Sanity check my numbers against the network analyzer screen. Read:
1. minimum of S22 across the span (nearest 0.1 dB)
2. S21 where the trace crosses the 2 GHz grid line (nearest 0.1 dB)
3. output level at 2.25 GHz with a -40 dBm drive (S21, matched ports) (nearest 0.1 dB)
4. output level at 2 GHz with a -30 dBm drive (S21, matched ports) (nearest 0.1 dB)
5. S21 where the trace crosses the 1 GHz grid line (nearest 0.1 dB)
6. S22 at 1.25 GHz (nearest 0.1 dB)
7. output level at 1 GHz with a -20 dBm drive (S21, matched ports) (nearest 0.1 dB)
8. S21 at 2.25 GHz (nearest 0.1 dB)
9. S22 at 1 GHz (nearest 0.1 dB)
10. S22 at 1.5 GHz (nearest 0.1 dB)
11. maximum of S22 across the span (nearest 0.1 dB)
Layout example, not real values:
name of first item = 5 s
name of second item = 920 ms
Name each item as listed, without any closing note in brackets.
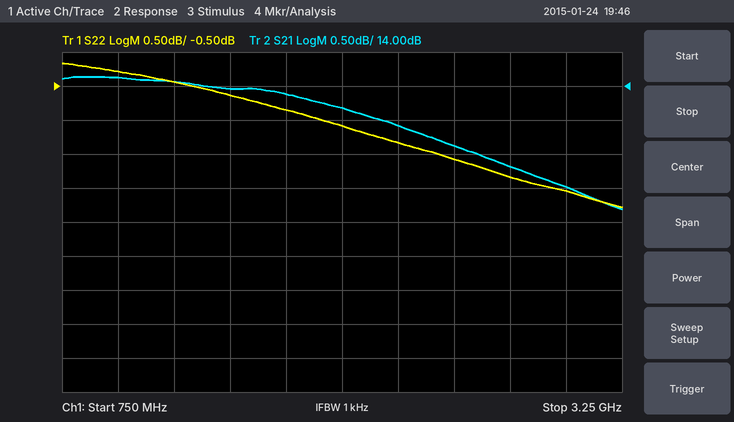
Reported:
minimum of S22 across the span = -2.3 dB
S21 where the trace crosses the 2 GHz grid line = 13.7 dB
output level at 2.25 GHz with a -40 dBm drive (S21, matched ports) = -26.6 dBm
output level at 2 GHz with a -30 dBm drive (S21, matched ports) = -16.3 dBm
S21 where the trace crosses the 1 GHz grid line = 14.1 dB
S22 at 1.25 GHz = -0.4 dB
output level at 1 GHz with a -20 dBm drive (S21, matched ports) = -5.9 dBm
S21 at 2.25 GHz = 13.4 dB
S22 at 1 GHz = -0.3 dB
S22 at 1.5 GHz = -0.6 dB
maximum of S22 across the span = -0.2 dB
